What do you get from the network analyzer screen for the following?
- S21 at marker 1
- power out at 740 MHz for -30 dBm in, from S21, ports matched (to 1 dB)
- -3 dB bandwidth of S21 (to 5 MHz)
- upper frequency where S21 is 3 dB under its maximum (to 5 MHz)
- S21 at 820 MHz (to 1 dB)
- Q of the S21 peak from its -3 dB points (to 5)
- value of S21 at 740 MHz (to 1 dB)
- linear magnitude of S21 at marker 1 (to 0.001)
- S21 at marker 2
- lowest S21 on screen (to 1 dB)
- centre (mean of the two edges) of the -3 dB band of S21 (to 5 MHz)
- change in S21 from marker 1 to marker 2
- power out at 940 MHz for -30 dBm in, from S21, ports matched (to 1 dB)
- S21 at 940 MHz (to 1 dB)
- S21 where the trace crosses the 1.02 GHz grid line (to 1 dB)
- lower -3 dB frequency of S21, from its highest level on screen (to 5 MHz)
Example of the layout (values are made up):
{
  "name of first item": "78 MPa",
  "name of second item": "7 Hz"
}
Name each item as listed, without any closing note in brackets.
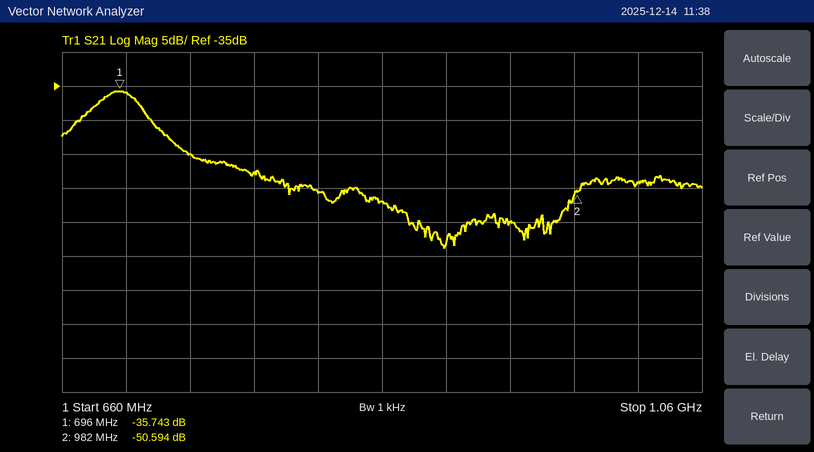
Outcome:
{
  "S21 at marker 1": "-35.743 dB",
  "power out at 740 MHz for -30 dBm in, from S21, ports matched": "-75 dBm",
  "-3 dB bandwidth of S21": "35 MHz",
  "upper frequency where S21 is 3 dB under its maximum": "710 MHz",
  "S21 at 820 MHz": "-51 dB",
  "Q of the S21 peak from its -3 dB points": "20",
  "value of S21 at 740 MHz": "-45 dB",
  "linear magnitude of S21 at marker 1": "0.016",
  "S21 at marker 2": "-50.594 dB",
  "lowest S21 on screen": "-59 dB",
  "centre (mean of the two edges) of the -3 dB band of S21": "695 MHz",
  "change in S21 from marker 1 to marker 2": "-14.851 dB",
  "power out at 940 MHz for -30 dBm in, from S21, ports matched": "-85 dBm",
  "S21 at 940 MHz": "-55 dB",
  "S21 where the trace crosses the 1.02 GHz grid line": "-49 dB",
  "lower -3 dB frequency of S21, from its highest level on screen": "675 MHz"
}
